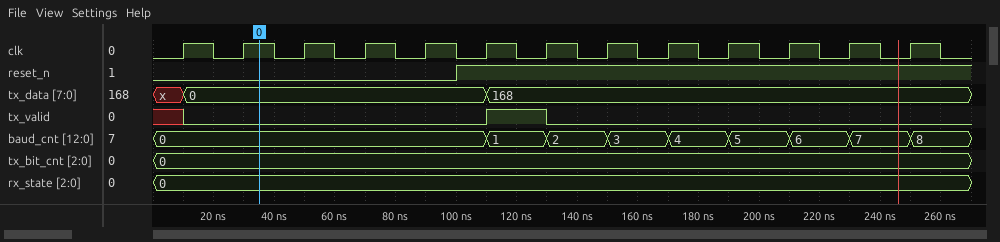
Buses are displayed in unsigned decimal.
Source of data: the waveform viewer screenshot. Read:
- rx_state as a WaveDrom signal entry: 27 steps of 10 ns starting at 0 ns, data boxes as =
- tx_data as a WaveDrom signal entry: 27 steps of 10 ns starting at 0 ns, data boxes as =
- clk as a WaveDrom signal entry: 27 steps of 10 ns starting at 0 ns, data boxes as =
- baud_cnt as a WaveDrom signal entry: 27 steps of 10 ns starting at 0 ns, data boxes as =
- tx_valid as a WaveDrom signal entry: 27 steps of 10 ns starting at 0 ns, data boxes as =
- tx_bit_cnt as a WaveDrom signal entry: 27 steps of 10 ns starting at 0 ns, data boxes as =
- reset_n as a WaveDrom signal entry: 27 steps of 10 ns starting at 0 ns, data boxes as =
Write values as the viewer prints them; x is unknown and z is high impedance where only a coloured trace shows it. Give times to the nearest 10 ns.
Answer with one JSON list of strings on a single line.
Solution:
["{name: 'rx_state', wave: '=..........................', data: '0'}", "{name: 'tx_data', wave: 'x=.........=...............', data: '0 168'}", "{name: 'clk', wave: '010101010101010101010101010'}", "{name: 'baud_cnt', wave: '=..........=.=.=.=.=.=.=.=.', data: '0 1 2 3 4 5 6 7 8'}", "{name: 'tx_valid', wave: 'x0.........1.0.............'}", "{name: 'tx_bit_cnt', wave: '=..........................', data: '0'}", "{name: 'reset_n', wave: '0.........1................'}"]
